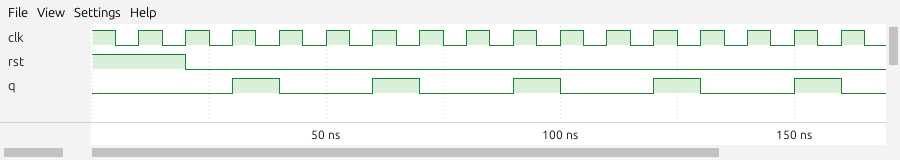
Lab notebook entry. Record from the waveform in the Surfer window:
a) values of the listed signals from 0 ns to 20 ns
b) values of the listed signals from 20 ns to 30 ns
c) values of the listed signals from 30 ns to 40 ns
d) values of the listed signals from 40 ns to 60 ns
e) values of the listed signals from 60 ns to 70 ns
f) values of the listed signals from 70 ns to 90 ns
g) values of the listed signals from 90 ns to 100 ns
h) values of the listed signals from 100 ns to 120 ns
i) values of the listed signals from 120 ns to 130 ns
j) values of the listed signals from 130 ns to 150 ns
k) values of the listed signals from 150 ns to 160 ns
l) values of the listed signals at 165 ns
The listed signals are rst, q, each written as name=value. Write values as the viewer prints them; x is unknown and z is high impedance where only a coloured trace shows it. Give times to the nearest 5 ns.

rst=1, q=0
rst=0, q=0
rst=0, q=1
rst=0, q=0
rst=0, q=1
rst=0, q=0
rst=0, q=1
rst=0, q=0
rst=0, q=1
rst=0, q=0
rst=0, q=1
rst=0, q=0
